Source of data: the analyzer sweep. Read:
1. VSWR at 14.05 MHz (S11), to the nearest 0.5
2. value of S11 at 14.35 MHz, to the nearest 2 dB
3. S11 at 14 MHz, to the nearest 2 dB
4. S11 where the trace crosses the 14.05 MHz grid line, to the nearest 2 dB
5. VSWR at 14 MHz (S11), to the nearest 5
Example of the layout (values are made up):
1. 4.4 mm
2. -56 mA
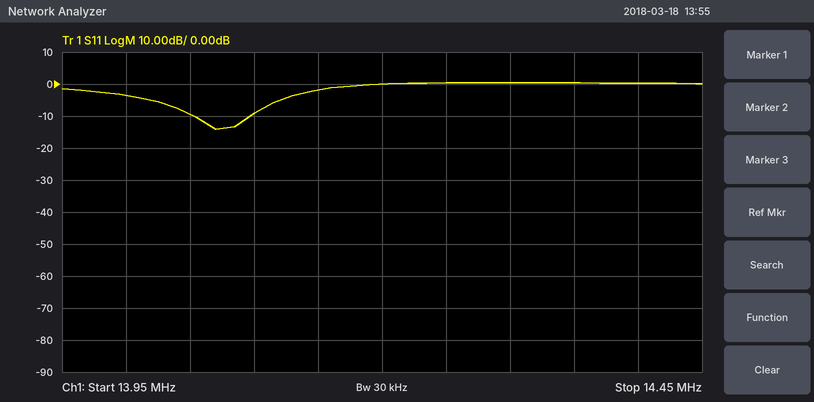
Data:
1. 2.0
2. 0 dB
3. -4 dB
4. -10 dB
5. 5
